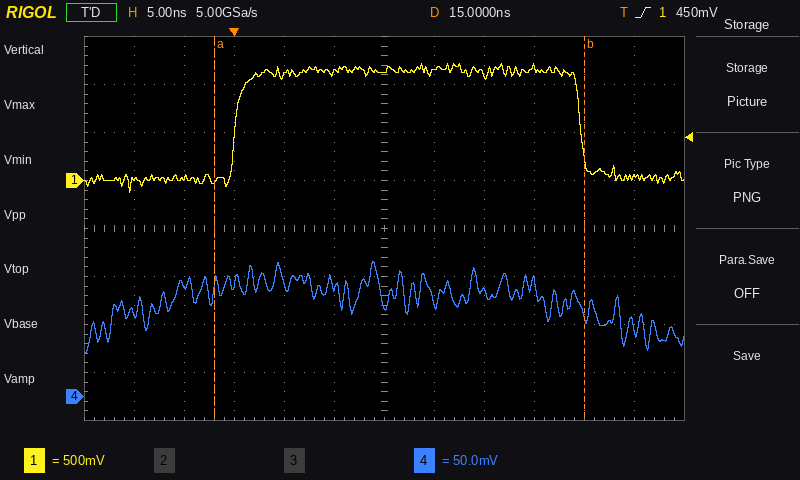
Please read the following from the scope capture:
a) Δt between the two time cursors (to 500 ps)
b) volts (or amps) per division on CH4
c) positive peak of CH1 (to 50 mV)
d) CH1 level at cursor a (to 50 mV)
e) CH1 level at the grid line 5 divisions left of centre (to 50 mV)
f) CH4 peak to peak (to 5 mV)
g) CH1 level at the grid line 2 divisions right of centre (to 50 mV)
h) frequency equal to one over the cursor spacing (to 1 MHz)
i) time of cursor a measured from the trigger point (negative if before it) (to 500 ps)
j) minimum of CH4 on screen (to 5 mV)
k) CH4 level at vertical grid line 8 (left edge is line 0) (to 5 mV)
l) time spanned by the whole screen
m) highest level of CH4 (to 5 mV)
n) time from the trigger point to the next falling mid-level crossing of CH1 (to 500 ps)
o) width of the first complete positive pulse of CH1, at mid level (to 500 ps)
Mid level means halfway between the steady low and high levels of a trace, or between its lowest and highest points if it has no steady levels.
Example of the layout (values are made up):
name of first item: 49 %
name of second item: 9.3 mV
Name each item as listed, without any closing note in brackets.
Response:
Δt between the two time cursors: 37.0 ns
volts (or amps) per division on CH4: 50 mV
positive peak of CH1: 1.20 V
CH1 level at cursor a: 0 mV
CH1 level at the grid line 5 divisions left of centre: 0 mV
CH4 peak to peak: 95 mV
CH1 level at the grid line 2 divisions right of centre: 1.10 V
frequency equal to one over the cursor spacing: 27 MHz
time of cursor a measured from the trigger point (negative if before it): -2.0 ns
minimum of CH4 on screen: 45 mV
CH4 level at vertical grid line 8 (left edge is line 0): 110 mV
time spanned by the whole screen: 60 ns
highest level of CH4: 140 mV
time from the trigger point to the next falling mid-level crossing of CH1: 34.5 ns
width of the first complete positive pulse of CH1, at mid level: 34.5 ns
